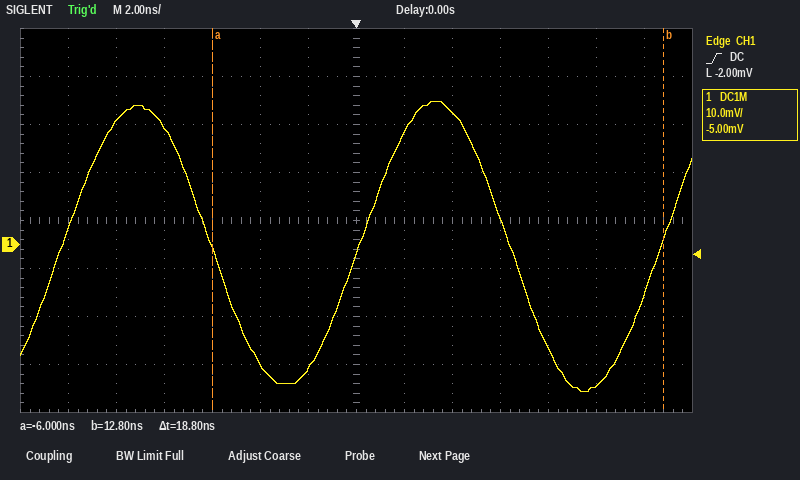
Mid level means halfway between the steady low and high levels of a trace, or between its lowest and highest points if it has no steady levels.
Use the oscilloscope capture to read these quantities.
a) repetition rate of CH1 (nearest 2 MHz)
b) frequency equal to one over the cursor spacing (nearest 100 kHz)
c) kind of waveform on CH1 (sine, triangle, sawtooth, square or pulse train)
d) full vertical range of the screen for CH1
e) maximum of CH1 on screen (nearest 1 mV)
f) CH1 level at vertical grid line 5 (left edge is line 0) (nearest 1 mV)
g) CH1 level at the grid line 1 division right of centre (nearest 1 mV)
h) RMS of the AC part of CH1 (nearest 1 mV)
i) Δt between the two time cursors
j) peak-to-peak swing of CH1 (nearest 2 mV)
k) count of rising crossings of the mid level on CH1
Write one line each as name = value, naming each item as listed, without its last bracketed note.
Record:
repetition rate of CH1 = 80 MHz
frequency equal to one over the cursor spacing = 53.2 MHz
kind of waveform on CH1 = sine
full vertical range of the screen for CH1 = 80 mV
maximum of CH1 on screen = 30 mV
CH1 level at vertical grid line 5 (left edge is line 0) = -25 mV
CH1 level at the grid line 1 division right of centre = 23 mV
RMS of the AC part of CH1 = 21 mV
Δt between the two time cursors = 18.8 ns
peak-to-peak swing of CH1 = 60 mV
count of rising crossings of the mid level on CH1 = 3
